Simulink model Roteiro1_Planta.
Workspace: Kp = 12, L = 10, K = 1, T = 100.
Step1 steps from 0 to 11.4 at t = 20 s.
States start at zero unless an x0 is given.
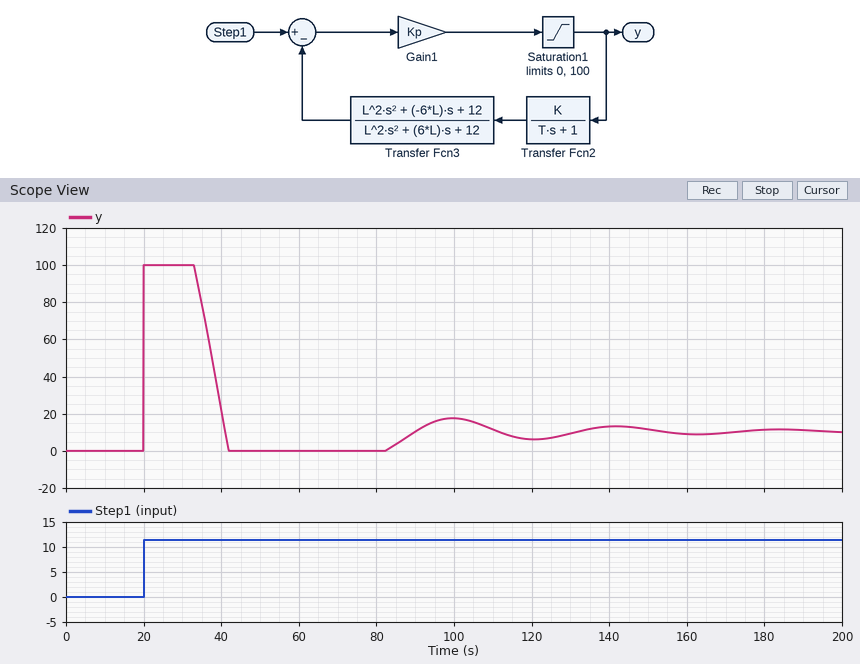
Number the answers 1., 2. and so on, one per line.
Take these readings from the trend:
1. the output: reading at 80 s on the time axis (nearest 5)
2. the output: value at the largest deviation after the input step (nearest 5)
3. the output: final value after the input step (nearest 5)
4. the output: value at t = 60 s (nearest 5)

1. 0
2. 100
3. 10
4. 0
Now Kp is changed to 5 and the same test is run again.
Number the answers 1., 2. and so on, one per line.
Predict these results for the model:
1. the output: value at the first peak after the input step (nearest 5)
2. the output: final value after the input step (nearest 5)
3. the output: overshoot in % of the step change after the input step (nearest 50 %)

1. 60
2. 10
3. 500 %
